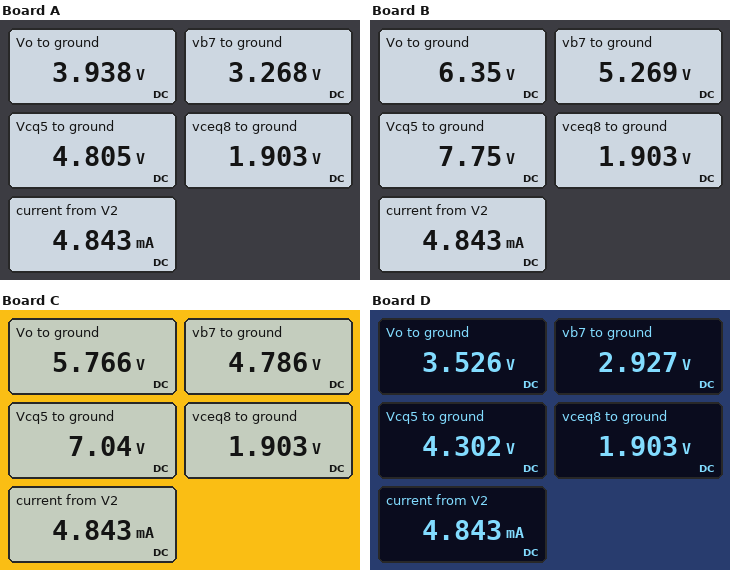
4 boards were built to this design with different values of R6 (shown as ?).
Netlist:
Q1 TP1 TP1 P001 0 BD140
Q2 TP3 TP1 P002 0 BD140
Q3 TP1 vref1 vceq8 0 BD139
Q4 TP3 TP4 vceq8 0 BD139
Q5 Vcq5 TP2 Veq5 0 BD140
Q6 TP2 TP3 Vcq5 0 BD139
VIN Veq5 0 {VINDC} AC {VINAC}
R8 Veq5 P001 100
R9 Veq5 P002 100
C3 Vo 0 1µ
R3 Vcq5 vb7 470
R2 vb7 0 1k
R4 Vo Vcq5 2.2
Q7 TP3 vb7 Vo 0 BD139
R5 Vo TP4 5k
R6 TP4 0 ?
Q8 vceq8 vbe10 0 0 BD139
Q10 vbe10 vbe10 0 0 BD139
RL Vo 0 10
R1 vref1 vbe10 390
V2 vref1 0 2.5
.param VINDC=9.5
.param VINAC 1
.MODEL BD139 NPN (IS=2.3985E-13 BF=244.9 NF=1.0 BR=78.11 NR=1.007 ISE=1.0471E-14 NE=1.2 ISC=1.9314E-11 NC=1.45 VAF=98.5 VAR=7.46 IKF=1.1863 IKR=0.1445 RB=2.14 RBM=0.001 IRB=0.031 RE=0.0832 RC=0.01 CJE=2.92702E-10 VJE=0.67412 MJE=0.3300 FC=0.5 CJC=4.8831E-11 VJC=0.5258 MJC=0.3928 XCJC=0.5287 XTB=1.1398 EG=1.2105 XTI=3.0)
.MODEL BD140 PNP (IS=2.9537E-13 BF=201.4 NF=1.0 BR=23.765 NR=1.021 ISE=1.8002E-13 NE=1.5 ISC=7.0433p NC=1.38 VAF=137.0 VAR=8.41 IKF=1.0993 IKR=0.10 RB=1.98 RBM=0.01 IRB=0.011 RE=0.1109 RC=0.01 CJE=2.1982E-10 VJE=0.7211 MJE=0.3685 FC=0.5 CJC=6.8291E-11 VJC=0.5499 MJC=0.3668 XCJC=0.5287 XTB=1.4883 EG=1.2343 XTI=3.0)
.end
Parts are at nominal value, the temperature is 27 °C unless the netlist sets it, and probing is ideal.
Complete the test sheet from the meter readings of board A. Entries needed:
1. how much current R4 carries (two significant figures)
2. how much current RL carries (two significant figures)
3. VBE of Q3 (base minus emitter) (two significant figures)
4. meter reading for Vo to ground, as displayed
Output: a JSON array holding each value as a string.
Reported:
["390 mA", "390 mA", "600 mV", "3.938 V"]
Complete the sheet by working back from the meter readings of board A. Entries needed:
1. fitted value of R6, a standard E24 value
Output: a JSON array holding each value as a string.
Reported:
["9.1 kΩ"]
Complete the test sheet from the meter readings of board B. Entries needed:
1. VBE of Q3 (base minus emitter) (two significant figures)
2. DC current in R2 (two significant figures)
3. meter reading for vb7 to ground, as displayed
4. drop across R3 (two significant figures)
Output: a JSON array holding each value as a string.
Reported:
["600 mV", "5.3 mA", "5.269 V", "2.5 V"]
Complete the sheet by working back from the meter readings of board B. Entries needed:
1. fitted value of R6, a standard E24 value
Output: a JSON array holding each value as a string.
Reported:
["3.3 kΩ"]
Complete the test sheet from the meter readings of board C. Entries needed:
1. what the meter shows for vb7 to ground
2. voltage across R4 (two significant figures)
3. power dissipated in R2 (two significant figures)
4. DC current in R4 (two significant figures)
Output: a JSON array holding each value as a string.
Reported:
["4.786 V", "1.3 V", "23 mW", "580 mA"]
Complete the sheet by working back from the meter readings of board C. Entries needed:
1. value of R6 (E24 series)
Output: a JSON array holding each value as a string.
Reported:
["3.9 kΩ"]
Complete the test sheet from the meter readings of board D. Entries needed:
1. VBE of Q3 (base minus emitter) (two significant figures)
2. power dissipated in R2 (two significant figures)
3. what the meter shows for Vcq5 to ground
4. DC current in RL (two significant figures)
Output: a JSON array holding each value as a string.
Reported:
["600 mV", "8.6 mW", "4.302 V", "350 mA"]
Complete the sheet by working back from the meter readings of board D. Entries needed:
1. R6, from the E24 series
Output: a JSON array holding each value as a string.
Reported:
["13 kΩ"]
